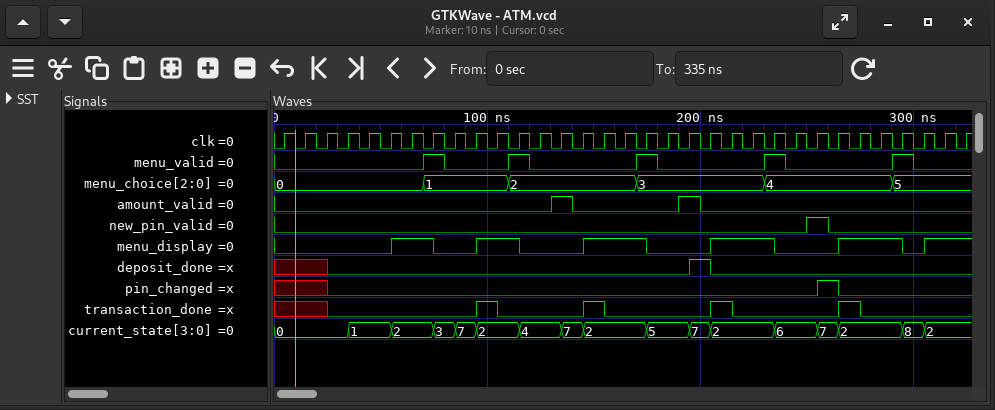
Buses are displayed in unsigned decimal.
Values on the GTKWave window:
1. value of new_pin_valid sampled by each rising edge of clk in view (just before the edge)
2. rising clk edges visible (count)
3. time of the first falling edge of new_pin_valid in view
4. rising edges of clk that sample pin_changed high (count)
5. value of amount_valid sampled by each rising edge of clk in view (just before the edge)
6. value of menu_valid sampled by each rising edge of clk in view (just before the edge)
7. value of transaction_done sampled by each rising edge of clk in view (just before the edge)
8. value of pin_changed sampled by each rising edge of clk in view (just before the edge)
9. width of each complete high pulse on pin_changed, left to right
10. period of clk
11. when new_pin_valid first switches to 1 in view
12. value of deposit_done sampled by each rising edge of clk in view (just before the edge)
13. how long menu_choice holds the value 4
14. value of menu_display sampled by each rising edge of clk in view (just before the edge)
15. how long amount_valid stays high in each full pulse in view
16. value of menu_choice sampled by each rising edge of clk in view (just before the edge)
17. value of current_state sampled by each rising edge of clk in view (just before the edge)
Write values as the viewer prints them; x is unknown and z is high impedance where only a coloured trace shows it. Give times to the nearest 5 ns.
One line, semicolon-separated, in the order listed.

0 0 0 0 0 0 0 0 0 0 0 0 0 0 0 0 0 0 0 0 0 0 0 0 0 1 0 0 0 0 0 0 0; 33; 260 ns; 1; 0 0 0 0 0 0 0 0 0 0 0 0 0 1 0 0 0 0 0 1 0 0 0 0 0 0 0 0 0 0 0 0 0; 0 0 0 0 0 0 0 1 0 0 0 1 0 0 0 0 0 1 0 0 0 0 0 1 0 0 0 0 0 1 0 0 0; x x x 0 0 0 0 0 0 0 1 0 0 0 0 1 0 0 0 0 0 1 0 0 0 0 0 1 0 0 0 0 0; x x x 0 0 0 0 0 0 0 0 0 0 0 0 0 0 0 0 0 0 0 0 0 0 0 1 0 0 0 0 0 0; 10 ns; 10 ns; 250 ns; x x x 0 0 0 0 0 0 0 0 0 0 0 0 0 0 0 0 0 1 0 0 0 0 0 0 0 0 0 0 0 0; 60 ns; 0 0 0 0 0 0 1 1 0 0 1 1 0 0 0 1 1 1 0 0 0 1 1 1 0 0 0 1 1 1 0 1 1; 10 ns, 10 ns; 0, 0, 0, 0, 0, 0, 0, 1, 1, 1, 1, 2, 2, 2, 2, 2, 2, 3, 3, 3, 3, 3, 3, 4, 4, 4, 4, 4, 4, 5, 5, 5, 5; 0, 0, 0, 0, 1, 1, 2, 2, 3, 7, 2, 2, 4, 4, 7, 2, 2, 2, 5, 5, 7, 2, 2, 2, 6, 6, 7, 2, 2, 2, 8, 2, 2
